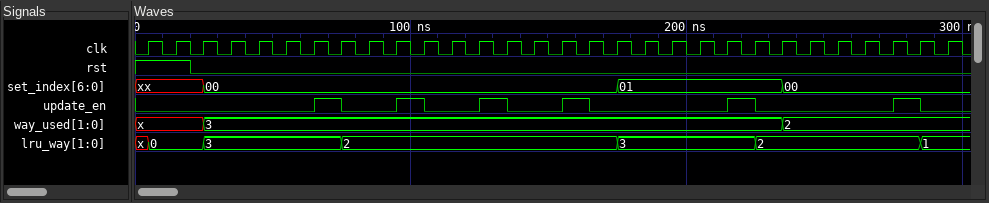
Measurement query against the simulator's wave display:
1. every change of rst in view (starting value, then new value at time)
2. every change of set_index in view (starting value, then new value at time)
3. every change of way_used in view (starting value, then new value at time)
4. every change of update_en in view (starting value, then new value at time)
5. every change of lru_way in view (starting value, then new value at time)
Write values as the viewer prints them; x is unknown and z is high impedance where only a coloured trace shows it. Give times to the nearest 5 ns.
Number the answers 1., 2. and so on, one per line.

1. 1, 0 at 20 ns
2. xx, 00 at 25 ns, 01 at 175 ns, 00 at 235 ns
3. x, 3 at 25 ns, 2 at 235 ns
4. 0, 1 at 65 ns, 0 at 75 ns, 1 at 95 ns, 0 at 105 ns, 1 at 125 ns, 0 at 135 ns, 1 at 155 ns, 0 at 165 ns, 1 at 215 ns, 0 at 225 ns, 1 at 275 ns, 0 at 285 ns
5. x, 0 at 5 ns, 3 at 25 ns, 2 at 75 ns, 3 at 175 ns, 2 at 225 ns, 1 at 285 ns
